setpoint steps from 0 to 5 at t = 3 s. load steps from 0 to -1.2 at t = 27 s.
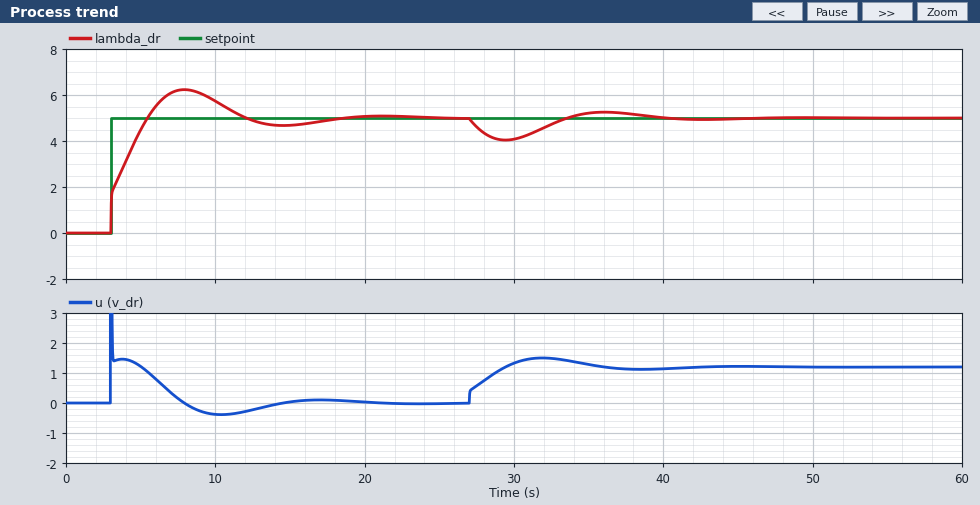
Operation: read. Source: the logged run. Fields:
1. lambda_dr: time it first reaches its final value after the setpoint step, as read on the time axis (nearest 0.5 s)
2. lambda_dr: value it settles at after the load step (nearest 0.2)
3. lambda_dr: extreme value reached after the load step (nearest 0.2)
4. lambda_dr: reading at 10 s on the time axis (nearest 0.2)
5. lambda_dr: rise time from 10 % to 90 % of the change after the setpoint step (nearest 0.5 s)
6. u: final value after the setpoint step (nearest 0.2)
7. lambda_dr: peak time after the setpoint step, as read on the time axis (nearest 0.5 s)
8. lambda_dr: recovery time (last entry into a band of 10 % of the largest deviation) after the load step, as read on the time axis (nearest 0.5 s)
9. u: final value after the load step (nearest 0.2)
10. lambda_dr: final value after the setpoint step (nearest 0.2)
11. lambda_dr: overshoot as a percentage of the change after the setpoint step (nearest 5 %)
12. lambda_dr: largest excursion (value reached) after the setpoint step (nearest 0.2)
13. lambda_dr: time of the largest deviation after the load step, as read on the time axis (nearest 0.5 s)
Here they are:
5.5 s
5.0
4.0
5.8
2.0 s
0.0
8.0 s
39.0 s
1.2
5.0
25 %
6.2
29.5 s
